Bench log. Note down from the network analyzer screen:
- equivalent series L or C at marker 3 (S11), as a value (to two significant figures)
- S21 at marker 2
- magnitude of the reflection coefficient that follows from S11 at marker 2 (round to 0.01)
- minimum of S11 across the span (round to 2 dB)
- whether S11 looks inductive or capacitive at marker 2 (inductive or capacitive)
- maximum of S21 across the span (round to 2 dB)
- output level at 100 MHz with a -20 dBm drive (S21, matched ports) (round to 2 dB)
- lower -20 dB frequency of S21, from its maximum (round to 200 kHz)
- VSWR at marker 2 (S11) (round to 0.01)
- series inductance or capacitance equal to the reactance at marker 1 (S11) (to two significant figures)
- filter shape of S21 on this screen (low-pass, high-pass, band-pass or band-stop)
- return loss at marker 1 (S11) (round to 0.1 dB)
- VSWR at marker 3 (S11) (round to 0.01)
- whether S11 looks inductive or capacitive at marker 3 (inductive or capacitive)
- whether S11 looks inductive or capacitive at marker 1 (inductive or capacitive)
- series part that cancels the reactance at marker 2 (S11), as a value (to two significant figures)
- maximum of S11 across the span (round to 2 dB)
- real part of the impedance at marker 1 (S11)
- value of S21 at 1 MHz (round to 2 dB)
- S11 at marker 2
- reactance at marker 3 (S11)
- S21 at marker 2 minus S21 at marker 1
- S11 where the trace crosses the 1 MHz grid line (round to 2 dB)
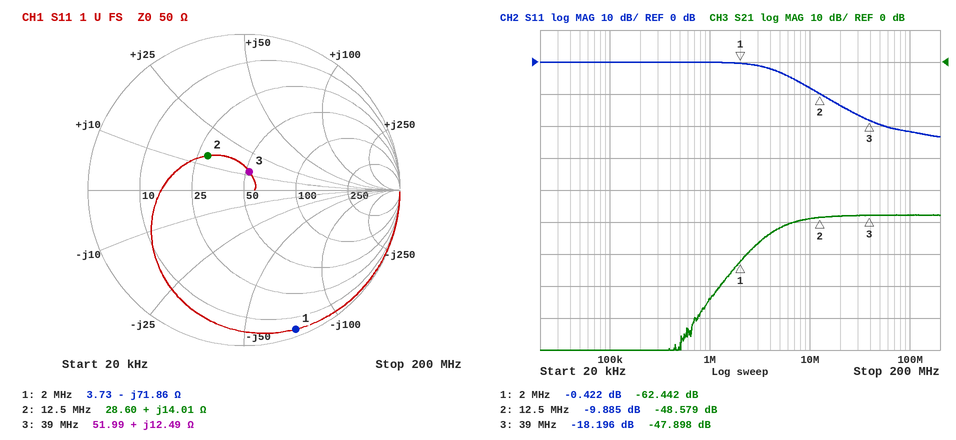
51 nH
-48.579 dB
0.32
-24 dB
inductive
-48 dB
-68 dBm
1.4 MHz
1.94
1.1 nF
high-pass
0.4 dB
1.28
inductive
capacitive
910 pF
0 dB
3.73 Ω
-74 dB
-9.885 dB
+12.49 Ω
13.863 dB
0 dB
